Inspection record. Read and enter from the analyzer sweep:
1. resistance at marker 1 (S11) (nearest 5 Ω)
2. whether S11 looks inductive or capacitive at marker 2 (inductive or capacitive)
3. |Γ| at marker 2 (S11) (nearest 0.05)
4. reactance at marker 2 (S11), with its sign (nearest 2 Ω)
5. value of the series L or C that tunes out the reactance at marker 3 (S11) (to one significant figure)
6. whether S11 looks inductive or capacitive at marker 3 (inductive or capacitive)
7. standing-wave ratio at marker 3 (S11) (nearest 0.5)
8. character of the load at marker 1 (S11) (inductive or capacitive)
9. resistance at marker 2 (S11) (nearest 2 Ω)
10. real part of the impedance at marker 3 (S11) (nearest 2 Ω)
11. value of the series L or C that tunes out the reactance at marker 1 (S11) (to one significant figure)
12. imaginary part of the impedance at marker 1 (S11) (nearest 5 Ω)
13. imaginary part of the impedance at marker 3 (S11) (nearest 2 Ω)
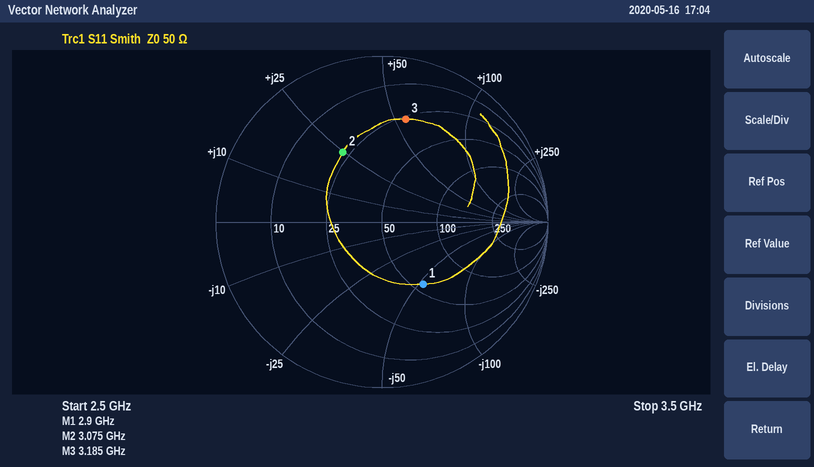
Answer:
55 Ω
inductive
0.50
+24 Ω
900 fF
inductive
4.5
capacitive
22 Ω
26 Ω
3 nH
-55 Ω
+56 Ω
